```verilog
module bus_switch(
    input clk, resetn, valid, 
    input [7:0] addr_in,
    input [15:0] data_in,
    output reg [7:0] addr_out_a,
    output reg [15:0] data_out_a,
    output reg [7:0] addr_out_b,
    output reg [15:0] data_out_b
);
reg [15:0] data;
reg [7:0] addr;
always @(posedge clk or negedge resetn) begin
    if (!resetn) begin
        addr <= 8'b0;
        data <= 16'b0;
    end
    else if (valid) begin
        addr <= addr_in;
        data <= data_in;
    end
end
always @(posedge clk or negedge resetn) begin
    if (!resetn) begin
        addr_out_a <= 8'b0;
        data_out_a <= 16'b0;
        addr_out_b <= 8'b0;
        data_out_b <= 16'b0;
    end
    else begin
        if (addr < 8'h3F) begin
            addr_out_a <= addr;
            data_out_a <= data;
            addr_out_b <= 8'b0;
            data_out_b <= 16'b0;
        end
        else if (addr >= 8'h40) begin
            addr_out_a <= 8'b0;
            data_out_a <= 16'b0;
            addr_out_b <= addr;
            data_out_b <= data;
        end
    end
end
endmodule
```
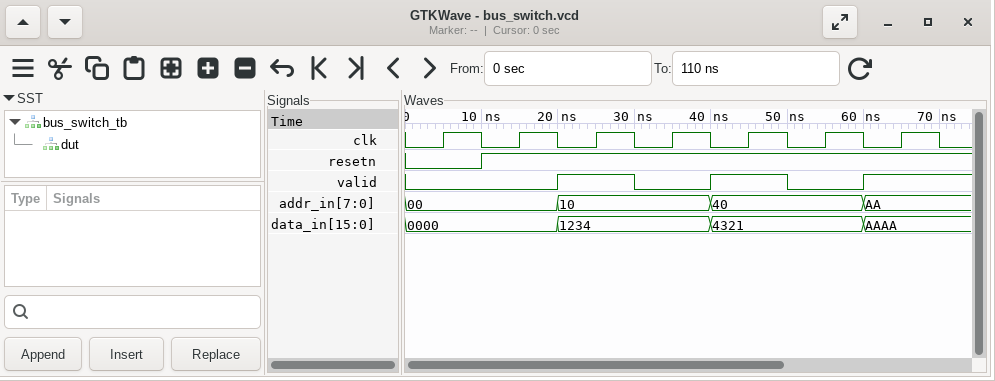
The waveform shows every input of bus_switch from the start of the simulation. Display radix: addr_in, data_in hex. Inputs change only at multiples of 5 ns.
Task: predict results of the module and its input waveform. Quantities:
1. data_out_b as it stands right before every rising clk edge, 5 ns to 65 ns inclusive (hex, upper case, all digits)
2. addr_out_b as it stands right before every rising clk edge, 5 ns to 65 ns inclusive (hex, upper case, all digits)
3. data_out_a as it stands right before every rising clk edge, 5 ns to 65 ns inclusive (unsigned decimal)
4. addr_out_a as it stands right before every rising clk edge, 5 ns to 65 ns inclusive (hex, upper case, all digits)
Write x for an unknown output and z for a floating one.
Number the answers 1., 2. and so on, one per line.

1. 0000, 0000, 0000, 0000, 0000, 0000, 4321
2. 00, 00, 00, 00, 00, 00, 40
3. 0, 0, 0, 0, 4660, 4660, 0
4. 00, 00, 00, 00, 10, 10, 00
